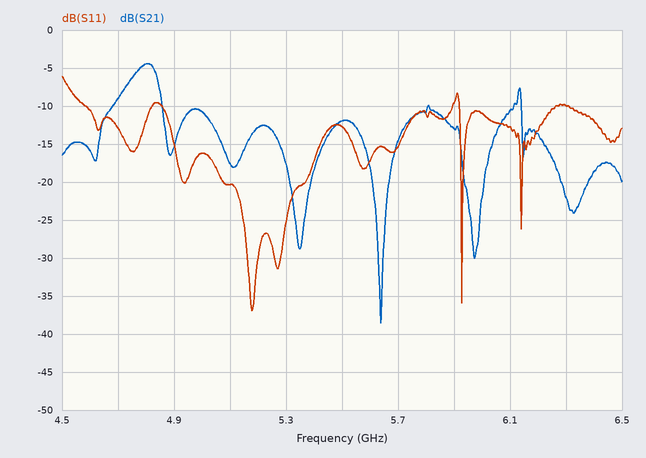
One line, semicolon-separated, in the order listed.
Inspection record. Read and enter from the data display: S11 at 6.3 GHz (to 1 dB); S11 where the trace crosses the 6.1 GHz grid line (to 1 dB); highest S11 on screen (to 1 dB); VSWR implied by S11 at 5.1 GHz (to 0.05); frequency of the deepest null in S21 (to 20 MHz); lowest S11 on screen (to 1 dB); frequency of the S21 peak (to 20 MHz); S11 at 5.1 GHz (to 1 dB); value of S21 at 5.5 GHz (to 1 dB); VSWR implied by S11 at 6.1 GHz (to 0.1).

-10 dB; -13 dB; -6 dB; 1.20; 5.64 GHz; -37 dB; 4.80 GHz; -20 dB; -12 dB; 1.6
